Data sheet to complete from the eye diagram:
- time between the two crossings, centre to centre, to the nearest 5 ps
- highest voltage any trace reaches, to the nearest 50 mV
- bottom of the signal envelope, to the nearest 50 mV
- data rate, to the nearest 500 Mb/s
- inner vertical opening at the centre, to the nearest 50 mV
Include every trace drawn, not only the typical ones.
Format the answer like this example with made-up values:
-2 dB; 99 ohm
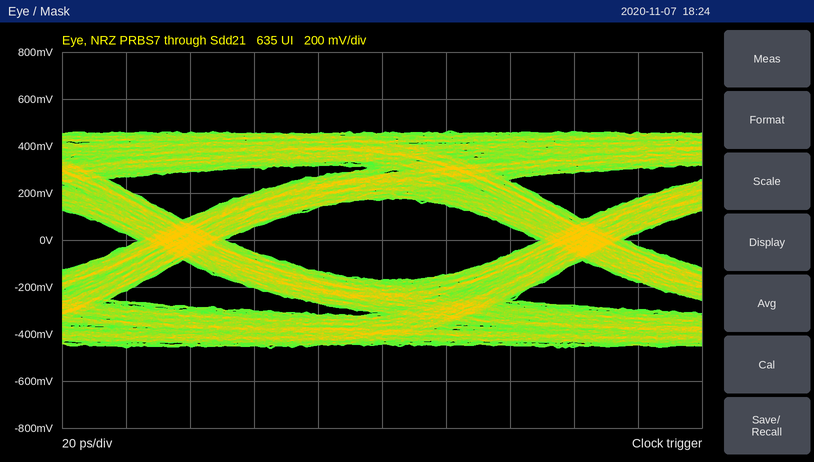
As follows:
125 ps; 450 mV; -450 mV; 8.0 Gb/s; 350 mV
